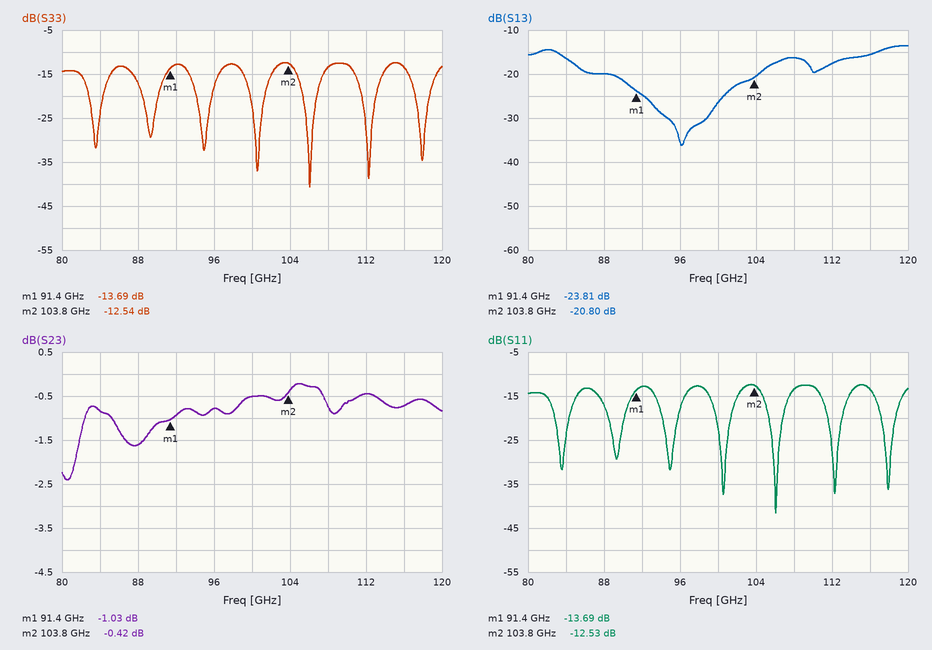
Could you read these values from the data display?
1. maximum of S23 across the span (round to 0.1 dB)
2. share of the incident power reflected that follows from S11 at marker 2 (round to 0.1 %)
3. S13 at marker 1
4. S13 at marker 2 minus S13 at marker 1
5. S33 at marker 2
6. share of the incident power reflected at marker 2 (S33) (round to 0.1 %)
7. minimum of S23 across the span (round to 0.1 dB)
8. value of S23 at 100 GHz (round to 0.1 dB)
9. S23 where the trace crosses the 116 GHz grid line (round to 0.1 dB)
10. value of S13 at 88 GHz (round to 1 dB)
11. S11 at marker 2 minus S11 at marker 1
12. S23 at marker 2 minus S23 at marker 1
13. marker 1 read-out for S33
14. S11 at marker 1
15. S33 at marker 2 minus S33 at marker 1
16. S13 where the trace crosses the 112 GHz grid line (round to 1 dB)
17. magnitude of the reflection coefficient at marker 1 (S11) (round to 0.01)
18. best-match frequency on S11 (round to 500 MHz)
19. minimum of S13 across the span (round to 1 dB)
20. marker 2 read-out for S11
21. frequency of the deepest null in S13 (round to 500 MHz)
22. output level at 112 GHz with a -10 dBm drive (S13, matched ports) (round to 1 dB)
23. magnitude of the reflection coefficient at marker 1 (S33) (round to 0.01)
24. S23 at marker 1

-0.2 dB
5.6 %
-23.81 dB
3.01 dB
-12.54 dB
5.6 %
-2.4 dB
-0.5 dB
-0.7 dB
-20 dB
1.16 dB
0.61 dB
-13.69 dB
-13.69 dB
1.15 dB
-18 dB
0.21
106.0 GHz
-36 dB
-12.53 dB
96.0 GHz
-28 dBm
0.21
-1.03 dB
